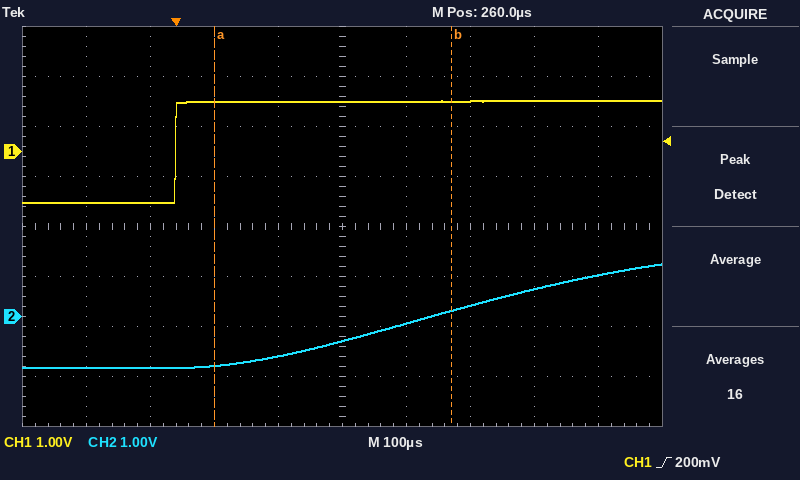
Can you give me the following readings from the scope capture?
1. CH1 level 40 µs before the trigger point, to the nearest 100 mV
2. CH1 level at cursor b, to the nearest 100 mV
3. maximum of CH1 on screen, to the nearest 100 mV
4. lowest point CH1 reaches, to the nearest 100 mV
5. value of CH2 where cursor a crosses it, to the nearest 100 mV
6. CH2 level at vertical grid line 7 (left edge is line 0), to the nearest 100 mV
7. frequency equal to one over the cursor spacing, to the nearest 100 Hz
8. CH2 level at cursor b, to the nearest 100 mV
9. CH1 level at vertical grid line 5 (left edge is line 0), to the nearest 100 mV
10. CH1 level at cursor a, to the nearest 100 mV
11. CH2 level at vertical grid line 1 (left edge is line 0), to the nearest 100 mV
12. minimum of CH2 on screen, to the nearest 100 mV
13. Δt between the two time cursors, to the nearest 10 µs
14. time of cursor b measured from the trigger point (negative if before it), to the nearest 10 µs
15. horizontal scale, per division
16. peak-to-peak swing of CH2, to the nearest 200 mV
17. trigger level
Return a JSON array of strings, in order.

["-1.0 V", "1.0 V", "1.0 V", "-1.0 V", "-1.0 V", "200 mV", "2.7 kHz", "100 mV", "1.0 V", "1.0 V", "-1.0 V", "-1.0 V", "370 µs", "+430 µs", "100 µs", "2.0 V", "200 mV"]
